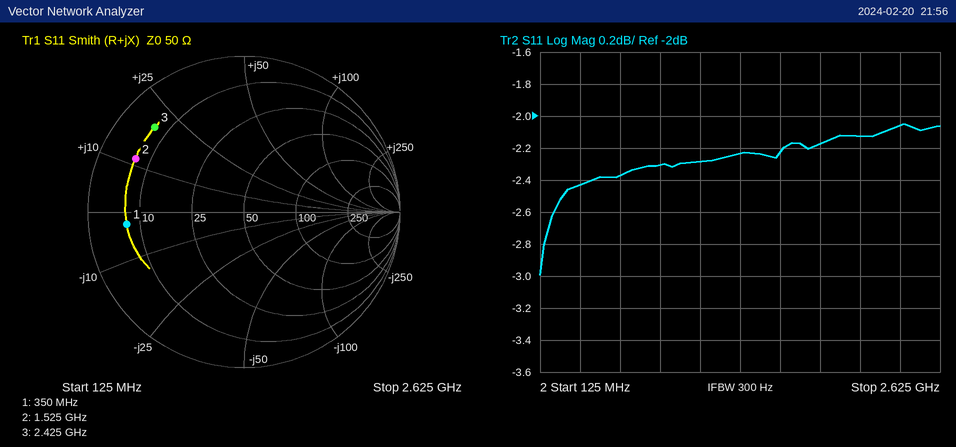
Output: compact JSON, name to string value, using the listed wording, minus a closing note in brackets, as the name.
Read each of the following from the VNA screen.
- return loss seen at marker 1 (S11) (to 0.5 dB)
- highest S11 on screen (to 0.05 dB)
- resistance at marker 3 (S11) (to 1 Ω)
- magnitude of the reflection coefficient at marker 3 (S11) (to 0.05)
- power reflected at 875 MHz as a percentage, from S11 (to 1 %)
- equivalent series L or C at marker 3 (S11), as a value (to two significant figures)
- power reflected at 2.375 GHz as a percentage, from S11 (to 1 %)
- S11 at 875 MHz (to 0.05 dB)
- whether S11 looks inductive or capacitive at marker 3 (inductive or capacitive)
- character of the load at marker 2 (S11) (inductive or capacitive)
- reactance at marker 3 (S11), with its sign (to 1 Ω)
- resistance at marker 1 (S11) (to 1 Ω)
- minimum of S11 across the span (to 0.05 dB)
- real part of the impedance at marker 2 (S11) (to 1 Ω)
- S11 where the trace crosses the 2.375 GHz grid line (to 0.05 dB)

{"return loss seen at marker 1 (S11)": "2.5 dB", "highest S11 on screen": "-2.05 dB", "resistance at marker 3 (S11)": "7 Ω", "magnitude of the reflection coefficient at marker 3 (S11)": "0.80", "power reflected at 875 MHz as a percentage, from S11": "59 %", "equivalent series L or C at marker 3 (S11), as a value": "1.3 nH", "power reflected at 2.375 GHz as a percentage, from S11": "62 %", "S11 at 875 MHz": "-2.30 dB", "whether S11 looks inductive or capacitive at marker 3": "inductive", "character of the load at marker 2 (S11)": "inductive", "reactance at marker 3 (S11), with its sign": "+20 Ω", "resistance at marker 1 (S11)": "7 Ω", "minimum of S11 across the span": "-3.00 dB", "real part of the impedance at marker 2 (S11)": "7 Ω", "S11 where the trace crosses the 2.375 GHz grid line": "-2.05 dB"}
